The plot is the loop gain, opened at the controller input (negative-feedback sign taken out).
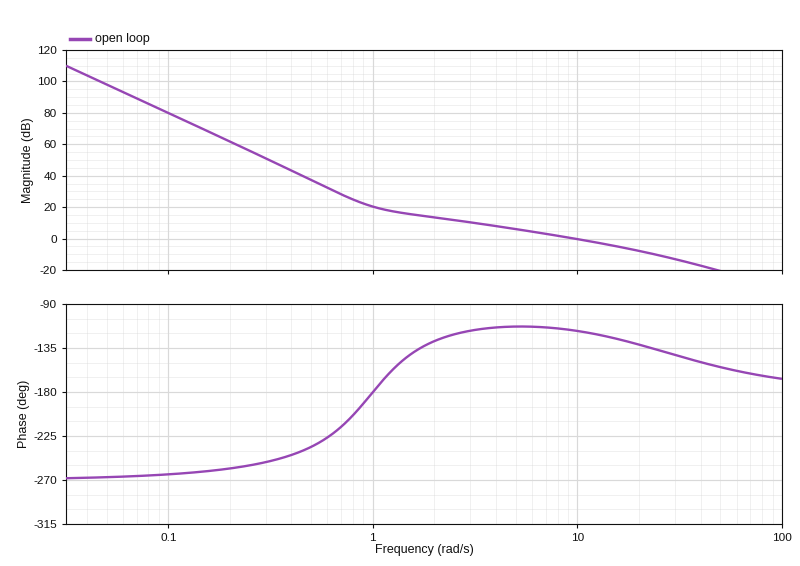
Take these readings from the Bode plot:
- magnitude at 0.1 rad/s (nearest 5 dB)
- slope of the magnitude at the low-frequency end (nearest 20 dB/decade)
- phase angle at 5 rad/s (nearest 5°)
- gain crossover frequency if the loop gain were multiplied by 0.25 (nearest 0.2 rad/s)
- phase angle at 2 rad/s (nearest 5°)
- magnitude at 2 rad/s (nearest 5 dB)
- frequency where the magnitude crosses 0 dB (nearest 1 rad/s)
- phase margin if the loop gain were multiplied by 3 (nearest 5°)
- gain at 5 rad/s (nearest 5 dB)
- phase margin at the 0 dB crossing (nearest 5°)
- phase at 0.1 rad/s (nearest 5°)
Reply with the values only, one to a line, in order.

80 dB
-60 dB/decade
-115°
2.4 rad/s
-130°
15 dB
10 rad/s
45°
5 dB
65°
-265°
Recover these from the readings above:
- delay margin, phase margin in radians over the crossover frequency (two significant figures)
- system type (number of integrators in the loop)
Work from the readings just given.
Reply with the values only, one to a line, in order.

0.11 s
3
